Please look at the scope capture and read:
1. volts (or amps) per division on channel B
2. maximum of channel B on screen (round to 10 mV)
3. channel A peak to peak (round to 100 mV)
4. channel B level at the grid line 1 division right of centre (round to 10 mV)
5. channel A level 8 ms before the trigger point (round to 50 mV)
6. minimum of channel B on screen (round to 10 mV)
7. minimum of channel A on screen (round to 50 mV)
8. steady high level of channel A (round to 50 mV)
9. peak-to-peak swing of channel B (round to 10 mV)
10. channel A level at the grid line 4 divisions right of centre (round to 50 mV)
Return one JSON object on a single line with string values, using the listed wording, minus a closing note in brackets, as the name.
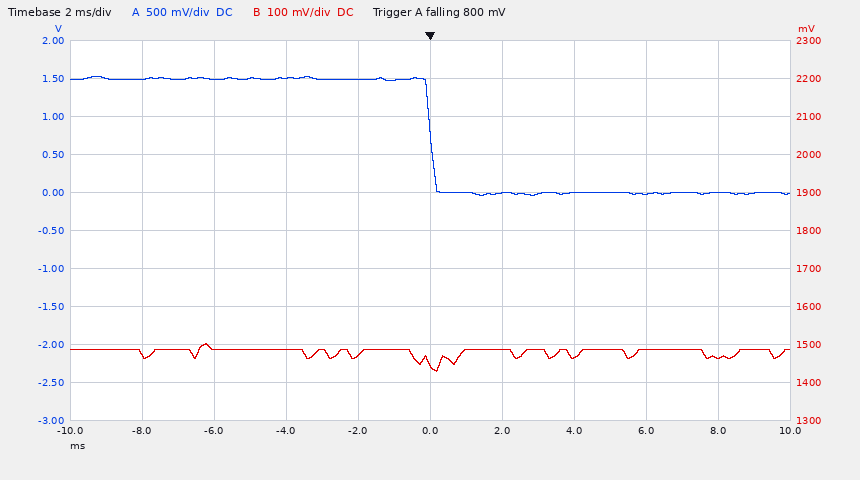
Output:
{"volts (or amps) per division on channel B": "100 mV", "maximum of channel B on screen": "1.50 V", "channel A peak to peak": "1.60 V", "channel B level at the grid line 1 division right of centre": "1.49 V", "channel A level 8 ms before the trigger point": "1.50 V", "minimum of channel B on screen": "1.43 V", "minimum of channel A on screen": "-50 mV", "steady high level of channel A": "1.50 V", "peak-to-peak swing of channel B": "70 mV", "channel A level at the grid line 4 divisions right of centre": "0 mV"}
